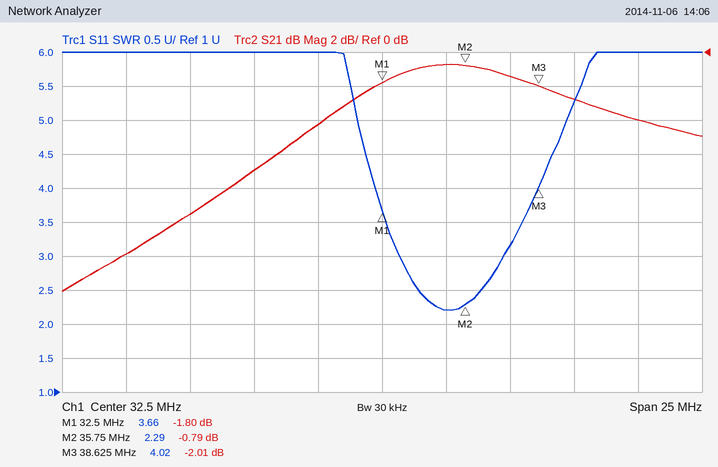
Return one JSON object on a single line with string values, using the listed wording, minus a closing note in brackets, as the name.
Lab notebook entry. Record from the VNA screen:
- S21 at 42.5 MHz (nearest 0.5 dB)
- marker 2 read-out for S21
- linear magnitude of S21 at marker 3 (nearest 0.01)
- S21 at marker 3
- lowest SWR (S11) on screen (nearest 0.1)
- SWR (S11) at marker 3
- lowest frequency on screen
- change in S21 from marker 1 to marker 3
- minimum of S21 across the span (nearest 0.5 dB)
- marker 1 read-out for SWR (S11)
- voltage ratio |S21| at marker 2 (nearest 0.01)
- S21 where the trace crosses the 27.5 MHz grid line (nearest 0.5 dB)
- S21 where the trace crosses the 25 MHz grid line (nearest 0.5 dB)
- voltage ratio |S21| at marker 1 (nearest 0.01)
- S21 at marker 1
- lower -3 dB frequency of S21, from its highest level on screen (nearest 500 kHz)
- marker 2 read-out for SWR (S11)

{"S21 at 42.5 MHz": "-4.0 dB", "marker 2 read-out for S21": "-0.79 dB", "linear magnitude of S21 at marker 3": "0.79", "S21 at marker 3": "-2.01 dB", "lowest SWR (S11) on screen": "2.2", "SWR (S11) at marker 3": "4.02", "lowest frequency on screen": "20 MHz", "change in S21 from marker 1 to marker 3": "-0.21 dB", "minimum of S21 across the span": "-14.0 dB", "marker 1 read-out for SWR": "3.66", "voltage ratio |S21| at marker 2": "0.91", "S21 where the trace crosses the 27.5 MHz grid line": "-7.0 dB", "S21 where the trace crosses the 25 MHz grid line": "-9.5 dB", "voltage ratio |S21| at marker 1": "0.81", "S21 at marker 1": "-1.80 dB", "lower -3 dB frequency of S21, from its highest level on screen": "30.5 MHz", "marker 2 read-out for SWR": "2.29"}
